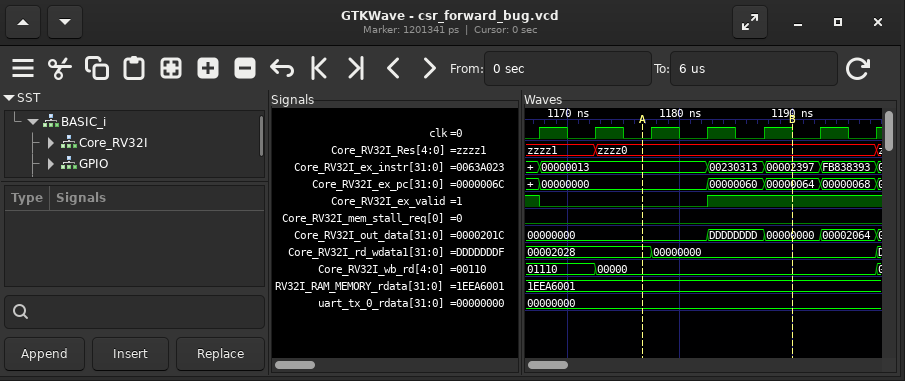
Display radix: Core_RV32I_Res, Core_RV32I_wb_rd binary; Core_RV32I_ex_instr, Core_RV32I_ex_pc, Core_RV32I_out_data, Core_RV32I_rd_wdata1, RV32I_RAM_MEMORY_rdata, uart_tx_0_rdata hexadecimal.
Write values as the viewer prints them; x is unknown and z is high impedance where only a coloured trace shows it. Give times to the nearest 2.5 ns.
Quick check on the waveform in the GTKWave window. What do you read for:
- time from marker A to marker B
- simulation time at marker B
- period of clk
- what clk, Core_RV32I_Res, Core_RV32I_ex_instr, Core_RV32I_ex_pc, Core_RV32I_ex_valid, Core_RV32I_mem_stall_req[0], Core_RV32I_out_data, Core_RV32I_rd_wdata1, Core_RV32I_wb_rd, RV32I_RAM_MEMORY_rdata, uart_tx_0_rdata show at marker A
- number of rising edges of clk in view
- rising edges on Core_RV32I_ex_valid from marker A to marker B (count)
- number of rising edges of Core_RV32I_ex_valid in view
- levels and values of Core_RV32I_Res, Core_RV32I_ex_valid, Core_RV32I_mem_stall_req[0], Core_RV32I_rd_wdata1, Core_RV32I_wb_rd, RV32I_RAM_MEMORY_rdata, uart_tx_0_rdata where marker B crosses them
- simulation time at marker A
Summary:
12.5 ns
1190 ns
5 ns
clk=0, Core_RV32I_Res=zzzz0, Core_RV32I_ex_instr=00000013, Core_RV32I_ex_pc=00000000, Core_RV32I_ex_valid=0, Core_RV32I_mem_stall_req[0]=0, Core_RV32I_out_data=00000000, Core_RV32I_rd_wdata1=00002028, Core_RV32I_wb_rd=00000, RV32I_RAM_MEMORY_rdata=1EEA6001, uart_tx_0_rdata=00000000
7
1
1
Core_RV32I_Res=zzzz0, Core_RV32I_ex_valid=1, Core_RV32I_mem_stall_req[0]=0, Core_RV32I_rd_wdata1=00000000, Core_RV32I_wb_rd=00000, RV32I_RAM_MEMORY_rdata=1EEA6001, uart_tx_0_rdata=00000000
1177.5 ns
